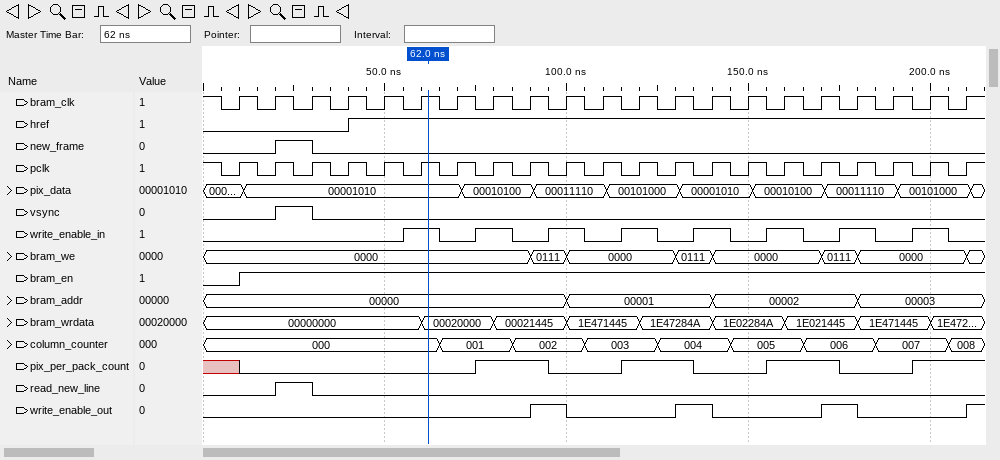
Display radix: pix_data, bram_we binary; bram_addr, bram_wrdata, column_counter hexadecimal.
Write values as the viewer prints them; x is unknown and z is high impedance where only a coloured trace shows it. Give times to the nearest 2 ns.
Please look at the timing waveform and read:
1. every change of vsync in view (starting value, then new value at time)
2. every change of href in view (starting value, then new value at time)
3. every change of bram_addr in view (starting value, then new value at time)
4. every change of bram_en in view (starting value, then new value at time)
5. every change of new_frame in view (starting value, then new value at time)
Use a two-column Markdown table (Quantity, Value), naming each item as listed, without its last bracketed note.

| Quantity | Value |
|---|---|
| every change of vsync in view | 0, 1 at 20 ns, 0 at 30 ns |
| every change of href in view | 0, 1 at 40 ns |
| every change of bram_addr in view | 00000, 00001 at 100 ns, 00002 at 140 ns, 00003 at 180 ns |
| every change of bram_en in view | 0, 1 at 10 ns |
| every change of new_frame in view | 0, 1 at 20 ns, 0 at 30 ns |
